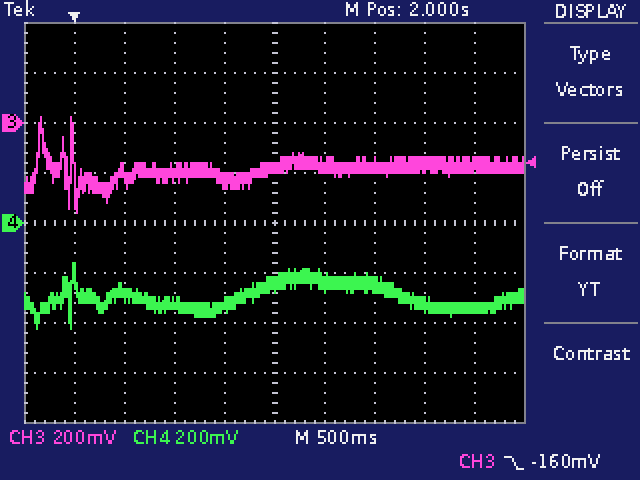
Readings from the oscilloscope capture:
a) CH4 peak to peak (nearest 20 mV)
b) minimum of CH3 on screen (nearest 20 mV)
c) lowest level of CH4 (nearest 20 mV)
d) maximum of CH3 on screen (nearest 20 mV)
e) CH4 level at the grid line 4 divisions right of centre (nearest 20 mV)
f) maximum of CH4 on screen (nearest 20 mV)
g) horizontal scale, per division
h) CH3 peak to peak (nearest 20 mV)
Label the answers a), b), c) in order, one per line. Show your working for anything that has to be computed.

a) -160 mV − (-420 mV) = 260 mV
b) -360 mV
c) -420 mV
d) 20 mV
e) -340 mV
f) -160 mV
g) 500 ms
h) 20 mV − (-360 mV) = 380 mV
